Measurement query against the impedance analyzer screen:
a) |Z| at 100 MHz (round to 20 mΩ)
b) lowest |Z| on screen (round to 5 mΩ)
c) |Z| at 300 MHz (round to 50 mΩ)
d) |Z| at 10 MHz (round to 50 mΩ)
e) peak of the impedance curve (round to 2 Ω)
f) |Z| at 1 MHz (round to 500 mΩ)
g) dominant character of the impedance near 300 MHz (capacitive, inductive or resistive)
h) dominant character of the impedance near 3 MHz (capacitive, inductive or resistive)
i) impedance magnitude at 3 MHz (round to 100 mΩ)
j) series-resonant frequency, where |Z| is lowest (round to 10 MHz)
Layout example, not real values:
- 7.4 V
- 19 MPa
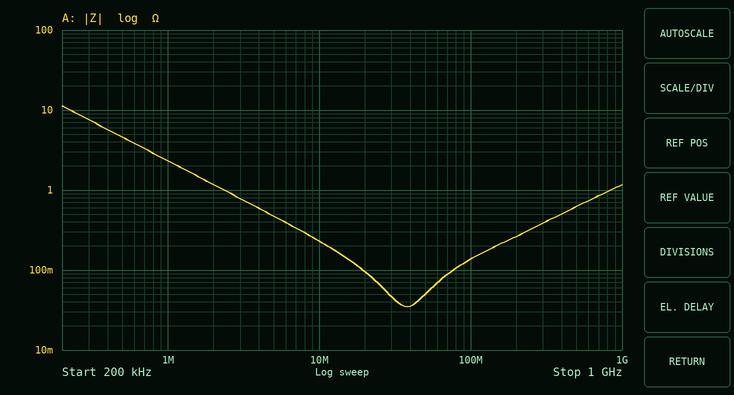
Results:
- 140 mΩ
- 35 mΩ
- 400 mΩ
- 250 mΩ
- 12 Ω
- 2.5 Ω
- inductive
- capacitive
- 800 mΩ
- 40 MHz
